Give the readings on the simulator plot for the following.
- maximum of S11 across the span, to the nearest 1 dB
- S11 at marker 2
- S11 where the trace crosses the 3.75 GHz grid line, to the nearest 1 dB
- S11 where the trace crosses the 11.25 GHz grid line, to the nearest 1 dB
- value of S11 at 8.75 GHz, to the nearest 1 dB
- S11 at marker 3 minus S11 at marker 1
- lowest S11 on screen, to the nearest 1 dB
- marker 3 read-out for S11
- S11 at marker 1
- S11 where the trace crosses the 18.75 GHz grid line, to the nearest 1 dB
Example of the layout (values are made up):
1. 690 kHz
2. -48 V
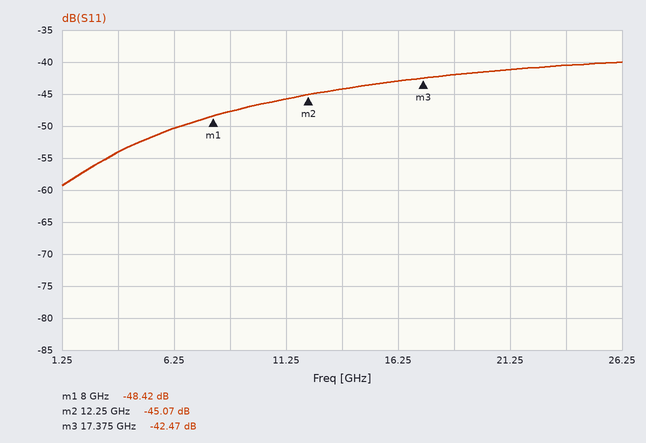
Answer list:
1. -40 dB
2. -45.07 dB
3. -54 dB
4. -46 dB
5. -48 dB
6. 5.95 dB
7. -59 dB
8. -42.47 dB
9. -48.42 dB
10. -42 dB
